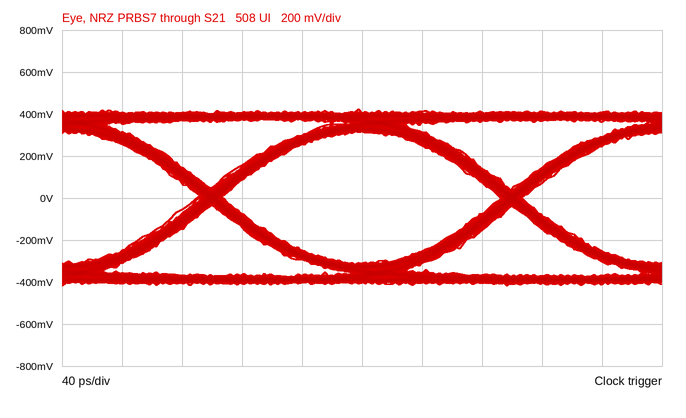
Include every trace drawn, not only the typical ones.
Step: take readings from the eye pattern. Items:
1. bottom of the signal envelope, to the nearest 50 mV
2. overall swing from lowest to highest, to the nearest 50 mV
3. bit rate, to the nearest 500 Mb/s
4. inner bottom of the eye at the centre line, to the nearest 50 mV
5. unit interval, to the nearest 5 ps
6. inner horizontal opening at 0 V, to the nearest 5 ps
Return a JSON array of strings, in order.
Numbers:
["-400 mV", "850 mV", "5.0 Gb/s", "-300 mV", "200 ps", "185 ps"]
